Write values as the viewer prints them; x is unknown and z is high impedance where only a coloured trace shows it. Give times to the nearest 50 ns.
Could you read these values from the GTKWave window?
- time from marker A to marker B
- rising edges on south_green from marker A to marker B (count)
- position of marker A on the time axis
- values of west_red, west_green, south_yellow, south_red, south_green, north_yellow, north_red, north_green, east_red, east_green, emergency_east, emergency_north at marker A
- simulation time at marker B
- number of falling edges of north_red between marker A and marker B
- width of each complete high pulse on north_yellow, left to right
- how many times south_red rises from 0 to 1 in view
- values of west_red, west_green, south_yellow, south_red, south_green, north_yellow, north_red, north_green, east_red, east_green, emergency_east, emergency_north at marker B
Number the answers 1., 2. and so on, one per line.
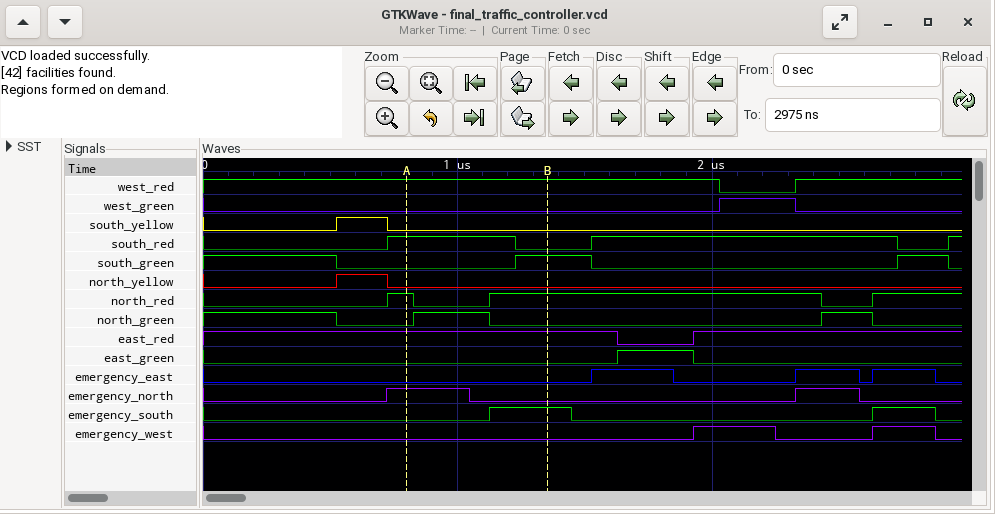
1. 550 ns
2. 1
3. 800 ns
4. west_red=1, west_green=0, south_yellow=0, south_red=1, south_green=0, north_yellow=0, north_red=1, north_green=0, east_red=1, east_green=0, emergency_east=0, emergency_north=1
5. 1350 ns
6. 1
7. 200 ns
8. 3
9. west_red=1, west_green=0, south_yellow=0, south_red=0, south_green=1, north_yellow=0, north_red=1, north_green=0, east_red=1, east_green=0, emergency_east=0, emergency_north=0
